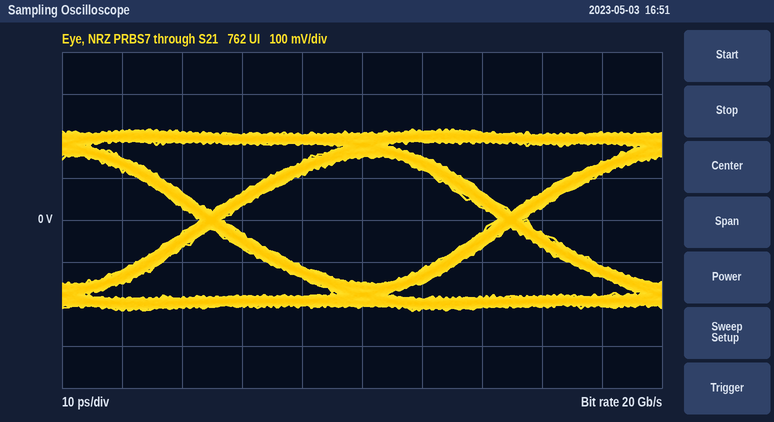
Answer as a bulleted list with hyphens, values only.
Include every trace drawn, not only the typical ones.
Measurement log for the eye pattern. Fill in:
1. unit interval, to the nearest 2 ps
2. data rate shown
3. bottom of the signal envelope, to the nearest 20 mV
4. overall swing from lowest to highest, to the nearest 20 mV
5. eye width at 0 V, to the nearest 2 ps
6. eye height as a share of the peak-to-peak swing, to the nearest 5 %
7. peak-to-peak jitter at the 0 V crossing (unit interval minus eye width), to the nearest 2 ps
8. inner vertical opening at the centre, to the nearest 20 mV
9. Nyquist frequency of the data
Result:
- 50 ps
- 20 Gb/s
- -220 mV
- 440 mV
- 46 ps
- 70 %
- 4 ps
- 300 mV
- 10 GHz
